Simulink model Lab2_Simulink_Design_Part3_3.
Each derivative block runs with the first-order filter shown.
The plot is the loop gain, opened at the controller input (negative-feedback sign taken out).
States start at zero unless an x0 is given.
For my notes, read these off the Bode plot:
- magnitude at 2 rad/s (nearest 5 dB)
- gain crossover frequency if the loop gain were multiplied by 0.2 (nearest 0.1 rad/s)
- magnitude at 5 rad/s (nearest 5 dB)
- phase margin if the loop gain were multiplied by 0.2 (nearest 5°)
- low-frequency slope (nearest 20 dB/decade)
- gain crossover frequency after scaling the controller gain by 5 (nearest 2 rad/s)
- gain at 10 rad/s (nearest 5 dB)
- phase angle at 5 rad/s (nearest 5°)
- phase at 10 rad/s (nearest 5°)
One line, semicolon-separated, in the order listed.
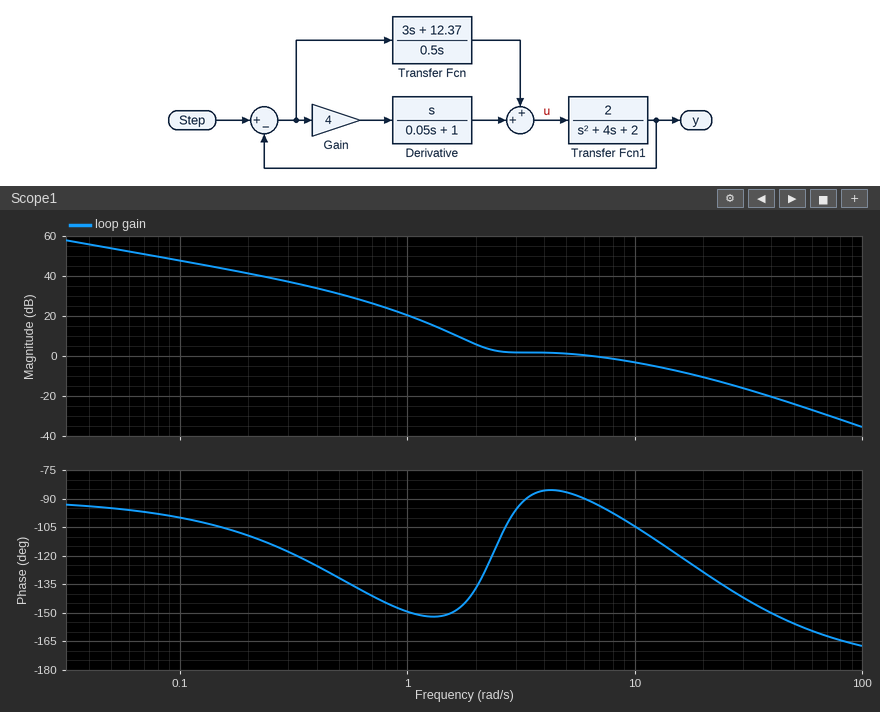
5 dB; 1.4 rad/s; 0 dB; 30°; -20 dB/decade; 26 rad/s; -5 dB; -85°; -105°
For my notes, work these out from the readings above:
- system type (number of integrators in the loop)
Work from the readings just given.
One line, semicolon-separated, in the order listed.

1
